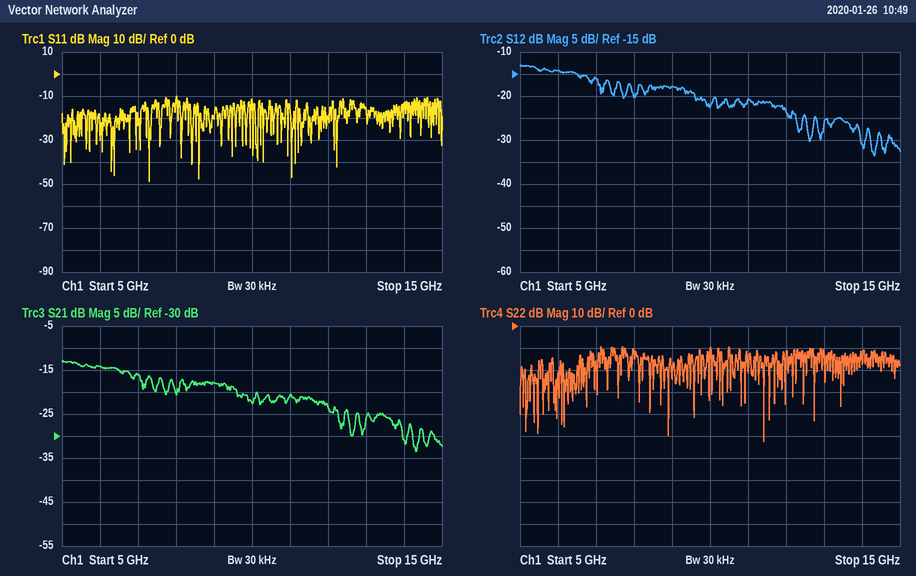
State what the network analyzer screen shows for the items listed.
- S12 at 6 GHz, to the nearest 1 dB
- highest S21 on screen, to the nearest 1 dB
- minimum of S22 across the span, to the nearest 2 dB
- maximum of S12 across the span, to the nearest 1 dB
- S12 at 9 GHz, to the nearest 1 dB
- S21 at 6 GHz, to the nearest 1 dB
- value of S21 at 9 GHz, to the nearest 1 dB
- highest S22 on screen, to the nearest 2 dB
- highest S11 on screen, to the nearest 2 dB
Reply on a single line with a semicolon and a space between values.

-14 dB; -13 dB; -52 dB; -13 dB; -18 dB; -14 dB; -18 dB; -10 dB; -10 dB
